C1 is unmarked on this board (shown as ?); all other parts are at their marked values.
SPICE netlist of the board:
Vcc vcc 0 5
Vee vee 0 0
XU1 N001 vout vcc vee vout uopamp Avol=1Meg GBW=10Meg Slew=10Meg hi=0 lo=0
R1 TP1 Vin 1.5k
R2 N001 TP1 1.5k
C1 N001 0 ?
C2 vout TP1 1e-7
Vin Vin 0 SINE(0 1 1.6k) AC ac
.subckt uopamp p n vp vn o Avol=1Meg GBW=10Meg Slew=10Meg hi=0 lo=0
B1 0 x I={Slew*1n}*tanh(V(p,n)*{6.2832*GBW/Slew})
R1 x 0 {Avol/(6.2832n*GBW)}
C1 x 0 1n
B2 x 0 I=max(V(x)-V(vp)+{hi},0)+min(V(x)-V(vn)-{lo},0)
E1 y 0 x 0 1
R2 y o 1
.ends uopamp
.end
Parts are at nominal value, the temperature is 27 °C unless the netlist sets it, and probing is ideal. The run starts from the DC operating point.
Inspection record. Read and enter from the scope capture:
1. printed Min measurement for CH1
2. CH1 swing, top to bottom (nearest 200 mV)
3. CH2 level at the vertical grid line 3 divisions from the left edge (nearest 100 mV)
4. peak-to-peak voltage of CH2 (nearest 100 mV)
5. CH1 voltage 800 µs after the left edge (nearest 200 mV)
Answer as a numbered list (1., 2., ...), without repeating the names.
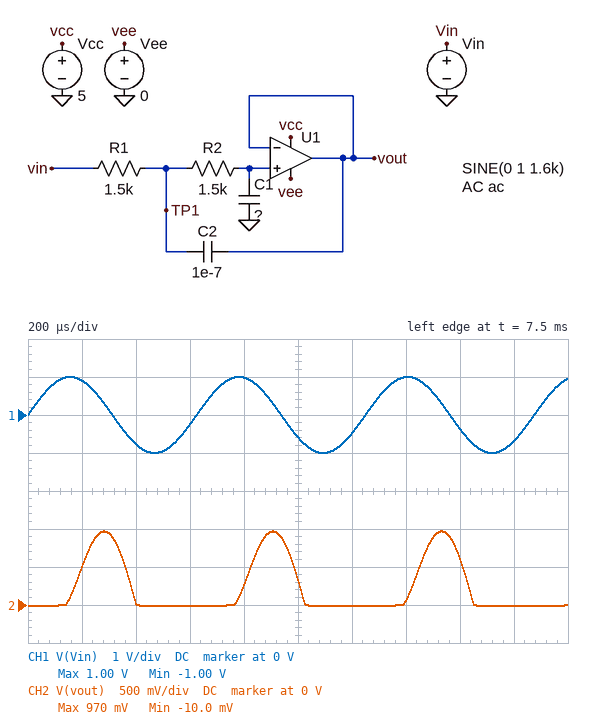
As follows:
1. -1.00 V
2. 2.0 V
3. 0 V
4. 1.0 V
5. 1.0 V
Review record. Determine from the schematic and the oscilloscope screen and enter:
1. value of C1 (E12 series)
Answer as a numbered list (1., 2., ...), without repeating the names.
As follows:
1. 18 nF
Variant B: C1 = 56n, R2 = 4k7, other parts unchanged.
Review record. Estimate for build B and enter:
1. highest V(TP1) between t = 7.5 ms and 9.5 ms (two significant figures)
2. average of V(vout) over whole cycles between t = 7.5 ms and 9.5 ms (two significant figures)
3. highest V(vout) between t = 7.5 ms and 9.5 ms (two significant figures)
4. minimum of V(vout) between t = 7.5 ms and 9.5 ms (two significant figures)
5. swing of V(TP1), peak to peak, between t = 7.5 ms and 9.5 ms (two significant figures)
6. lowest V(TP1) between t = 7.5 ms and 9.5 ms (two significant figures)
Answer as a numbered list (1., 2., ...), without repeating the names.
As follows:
1. 540 mV
2. 59 mV
3. 200 mV
4. -7.7 mV
5. 1.1 V
6. -570 mV
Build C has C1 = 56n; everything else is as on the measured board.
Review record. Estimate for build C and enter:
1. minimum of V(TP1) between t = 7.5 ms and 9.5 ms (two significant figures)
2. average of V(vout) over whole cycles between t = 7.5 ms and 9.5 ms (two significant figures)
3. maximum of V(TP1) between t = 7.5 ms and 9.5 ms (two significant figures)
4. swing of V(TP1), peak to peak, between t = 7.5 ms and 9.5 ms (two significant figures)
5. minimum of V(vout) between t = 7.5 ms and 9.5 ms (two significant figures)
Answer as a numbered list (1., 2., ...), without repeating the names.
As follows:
1. -500 mV
2. 130 mV
3. 590 mV
4. 1.1 V
5. -9.6 mV
